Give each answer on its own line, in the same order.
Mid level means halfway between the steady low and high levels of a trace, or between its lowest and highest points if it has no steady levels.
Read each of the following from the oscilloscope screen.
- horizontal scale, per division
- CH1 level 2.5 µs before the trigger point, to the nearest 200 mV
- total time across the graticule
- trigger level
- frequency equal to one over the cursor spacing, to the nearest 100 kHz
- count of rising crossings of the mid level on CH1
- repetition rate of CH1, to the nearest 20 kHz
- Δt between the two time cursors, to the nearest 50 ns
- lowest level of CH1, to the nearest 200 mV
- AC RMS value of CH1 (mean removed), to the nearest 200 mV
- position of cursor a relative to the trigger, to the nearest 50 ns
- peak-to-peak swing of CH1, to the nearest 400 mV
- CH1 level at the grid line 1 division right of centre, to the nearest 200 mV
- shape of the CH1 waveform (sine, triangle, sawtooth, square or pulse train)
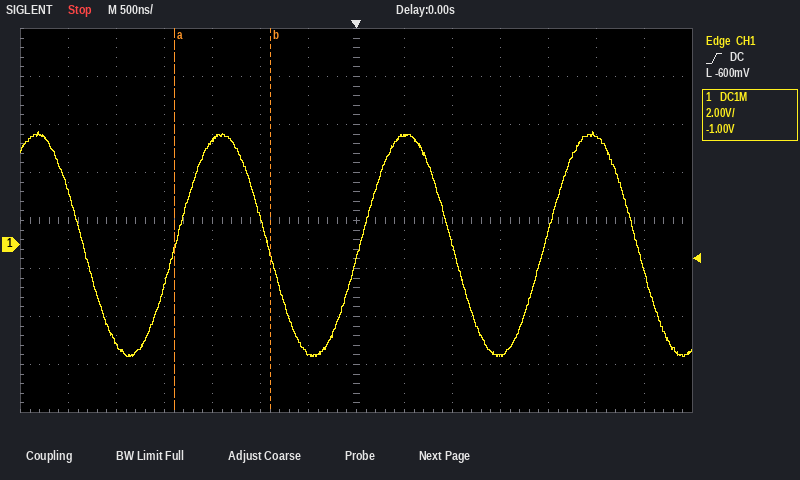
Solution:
500 ns
-4.2 V
7 µs
-600 mV
1.0 MHz
3
520 kHz
1.00 µs
-4.6 V
3.2 V
-1.90 µs
9.2 V
4.6 V
sine
